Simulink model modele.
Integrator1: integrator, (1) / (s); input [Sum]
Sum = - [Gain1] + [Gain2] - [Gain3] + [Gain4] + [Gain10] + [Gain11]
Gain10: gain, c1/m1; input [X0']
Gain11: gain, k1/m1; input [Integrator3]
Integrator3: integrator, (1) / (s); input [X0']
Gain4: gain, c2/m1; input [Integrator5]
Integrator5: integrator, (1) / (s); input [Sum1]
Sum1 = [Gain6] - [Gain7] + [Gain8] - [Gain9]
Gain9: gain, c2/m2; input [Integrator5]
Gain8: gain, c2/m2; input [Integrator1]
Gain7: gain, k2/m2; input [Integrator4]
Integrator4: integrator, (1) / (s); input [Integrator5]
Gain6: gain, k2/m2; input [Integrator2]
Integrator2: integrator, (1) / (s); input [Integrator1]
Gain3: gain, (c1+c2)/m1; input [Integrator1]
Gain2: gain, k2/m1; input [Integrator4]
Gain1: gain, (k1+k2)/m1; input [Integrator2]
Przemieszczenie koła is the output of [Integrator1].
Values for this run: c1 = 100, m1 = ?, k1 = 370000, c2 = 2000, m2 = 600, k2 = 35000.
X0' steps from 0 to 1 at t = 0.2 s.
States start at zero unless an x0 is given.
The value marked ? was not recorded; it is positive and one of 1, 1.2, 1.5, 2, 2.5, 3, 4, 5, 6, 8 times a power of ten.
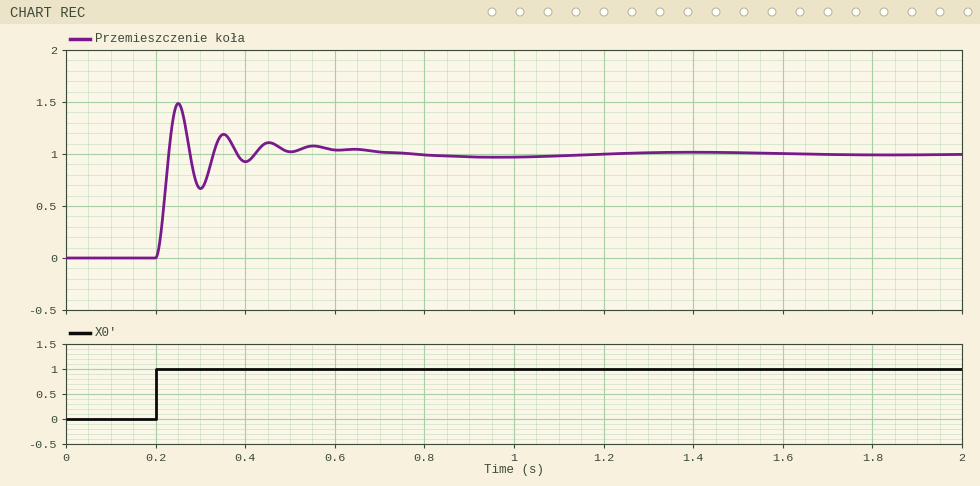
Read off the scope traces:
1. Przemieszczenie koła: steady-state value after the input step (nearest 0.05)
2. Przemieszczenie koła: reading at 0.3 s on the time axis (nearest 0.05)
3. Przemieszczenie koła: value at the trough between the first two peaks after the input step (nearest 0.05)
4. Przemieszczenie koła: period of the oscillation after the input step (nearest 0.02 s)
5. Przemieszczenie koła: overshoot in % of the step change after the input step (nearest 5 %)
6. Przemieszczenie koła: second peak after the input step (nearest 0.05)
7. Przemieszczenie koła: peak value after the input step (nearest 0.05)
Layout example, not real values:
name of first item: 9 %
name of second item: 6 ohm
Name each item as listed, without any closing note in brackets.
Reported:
Przemieszczenie koła: steady-state value after the input step: 1.00
Przemieszczenie koła: reading at 0.3 s on the time axis: 0.65
Przemieszczenie koła: value at the trough between the first two peaks after the input step: 0.65
Przemieszczenie koła: period of the oscillation after the input step: 0.10 s
Przemieszczenie koła: overshoot in % of the step change after the input step: 50 %
Przemieszczenie koła: second peak after the input step: 1.20
Przemieszczenie koła: peak value after the input step: 1.50
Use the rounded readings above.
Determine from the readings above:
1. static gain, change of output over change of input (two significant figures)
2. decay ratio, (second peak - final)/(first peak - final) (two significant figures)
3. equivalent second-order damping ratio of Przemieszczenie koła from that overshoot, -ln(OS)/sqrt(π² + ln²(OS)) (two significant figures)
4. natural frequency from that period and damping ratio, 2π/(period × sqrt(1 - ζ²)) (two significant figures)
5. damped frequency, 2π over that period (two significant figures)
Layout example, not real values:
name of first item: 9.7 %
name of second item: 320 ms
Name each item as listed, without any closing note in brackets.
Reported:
static gain, change of output over change of input: 1.0
decay ratio, (second peak - final)/(first peak - final): 0.40
equivalent second-order damping ratio of Przemieszczenie koła from that overshoot, -ln(OS)/sqrt(π² + ln²(OS)): 0.22
natural frequency from that period and damping ratio, 2π/(period × sqrt(1 - ζ²)): 64 rad/s
damped frequency, 2π over that period: 63 rad/s
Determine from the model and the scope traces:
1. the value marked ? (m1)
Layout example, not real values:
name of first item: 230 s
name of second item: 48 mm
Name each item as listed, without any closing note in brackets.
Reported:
the value marked ?: 100
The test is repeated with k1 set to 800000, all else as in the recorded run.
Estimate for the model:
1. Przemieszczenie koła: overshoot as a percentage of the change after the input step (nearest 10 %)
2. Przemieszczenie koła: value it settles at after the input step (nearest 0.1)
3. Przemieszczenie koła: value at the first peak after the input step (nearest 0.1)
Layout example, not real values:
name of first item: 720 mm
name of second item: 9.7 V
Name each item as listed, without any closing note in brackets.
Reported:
Przemieszczenie koła: overshoot as a percentage of the change after the input step: 60 %
Przemieszczenie koła: value it settles at after the input step: 1.0
Przemieszczenie koła: value at the first peak after the input step: 1.6
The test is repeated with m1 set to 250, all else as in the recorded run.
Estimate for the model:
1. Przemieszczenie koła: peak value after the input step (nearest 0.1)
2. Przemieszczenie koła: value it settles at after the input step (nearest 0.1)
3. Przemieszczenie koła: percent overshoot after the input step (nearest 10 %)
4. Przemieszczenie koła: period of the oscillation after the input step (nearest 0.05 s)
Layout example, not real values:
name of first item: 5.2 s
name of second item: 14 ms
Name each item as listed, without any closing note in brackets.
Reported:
Przemieszczenie koła: peak value after the input step: 1.6
Przemieszczenie koła: value it settles at after the input step: 1.0
Przemieszczenie koła: percent overshoot after the input step: 60 %
Przemieszczenie koła: period of the oscillation after the input step: 0.15 s
